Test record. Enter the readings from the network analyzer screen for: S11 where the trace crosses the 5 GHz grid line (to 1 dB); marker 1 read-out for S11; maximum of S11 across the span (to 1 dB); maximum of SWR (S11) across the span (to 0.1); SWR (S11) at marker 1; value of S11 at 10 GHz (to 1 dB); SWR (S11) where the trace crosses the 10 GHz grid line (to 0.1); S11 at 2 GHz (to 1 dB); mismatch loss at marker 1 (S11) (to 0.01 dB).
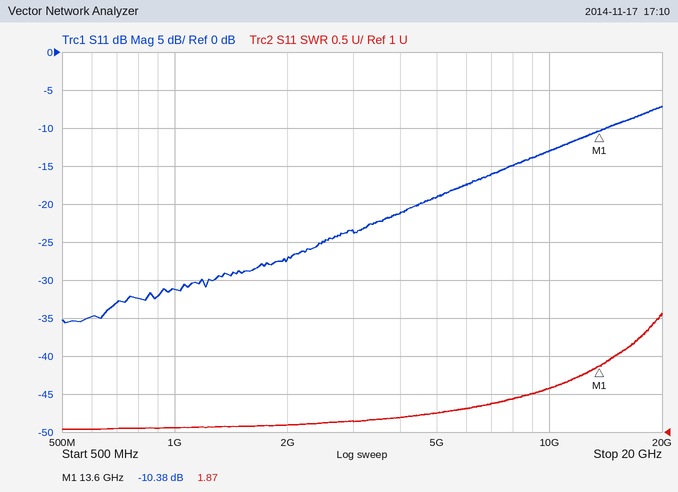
-19 dB
-10.38 dB
-7 dB
2.6
1.87
-13 dB
1.6
-27 dB
0.42 dB
